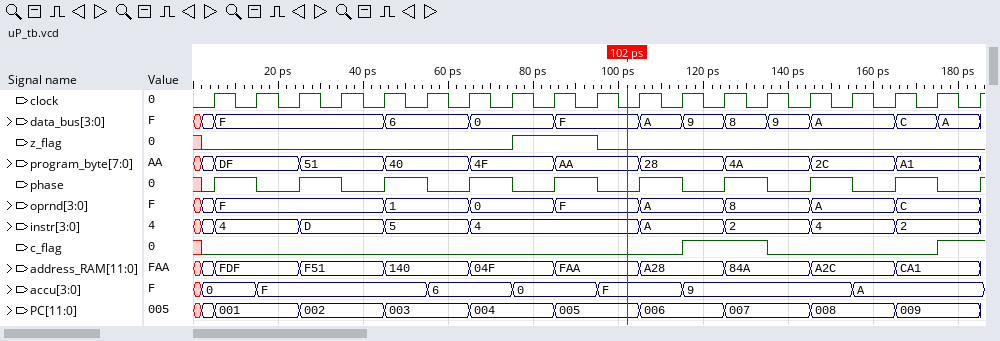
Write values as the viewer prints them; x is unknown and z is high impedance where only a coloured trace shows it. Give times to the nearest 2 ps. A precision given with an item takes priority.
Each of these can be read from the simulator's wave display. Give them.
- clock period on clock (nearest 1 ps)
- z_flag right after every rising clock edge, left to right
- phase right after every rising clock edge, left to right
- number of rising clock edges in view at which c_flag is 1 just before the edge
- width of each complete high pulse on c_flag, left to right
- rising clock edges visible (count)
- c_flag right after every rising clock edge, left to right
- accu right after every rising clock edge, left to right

10 ps
0 0 0 0 0 0 0 1 1 0 0 0 0 0 0 0 0 0 0
1 0 1 0 1 0 1 0 1 0 1 0 1 0 1 0 1 0 1
3
20 ps
19
0 0 0 0 0 0 0 0 0 0 0 1 1 0 0 0 0 1 1
0, F, F, F, F, 6, 6, 0, 0, F, F, 9, 9, 9, 9, A, A, A, A
